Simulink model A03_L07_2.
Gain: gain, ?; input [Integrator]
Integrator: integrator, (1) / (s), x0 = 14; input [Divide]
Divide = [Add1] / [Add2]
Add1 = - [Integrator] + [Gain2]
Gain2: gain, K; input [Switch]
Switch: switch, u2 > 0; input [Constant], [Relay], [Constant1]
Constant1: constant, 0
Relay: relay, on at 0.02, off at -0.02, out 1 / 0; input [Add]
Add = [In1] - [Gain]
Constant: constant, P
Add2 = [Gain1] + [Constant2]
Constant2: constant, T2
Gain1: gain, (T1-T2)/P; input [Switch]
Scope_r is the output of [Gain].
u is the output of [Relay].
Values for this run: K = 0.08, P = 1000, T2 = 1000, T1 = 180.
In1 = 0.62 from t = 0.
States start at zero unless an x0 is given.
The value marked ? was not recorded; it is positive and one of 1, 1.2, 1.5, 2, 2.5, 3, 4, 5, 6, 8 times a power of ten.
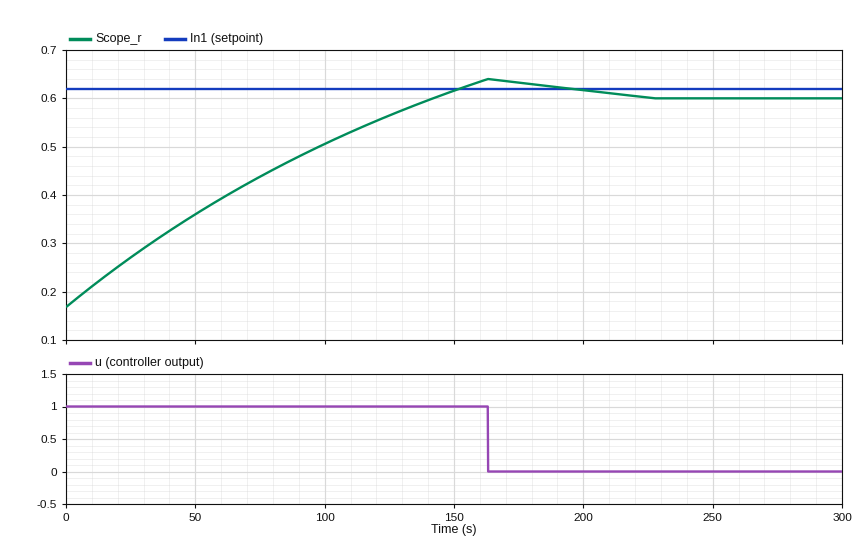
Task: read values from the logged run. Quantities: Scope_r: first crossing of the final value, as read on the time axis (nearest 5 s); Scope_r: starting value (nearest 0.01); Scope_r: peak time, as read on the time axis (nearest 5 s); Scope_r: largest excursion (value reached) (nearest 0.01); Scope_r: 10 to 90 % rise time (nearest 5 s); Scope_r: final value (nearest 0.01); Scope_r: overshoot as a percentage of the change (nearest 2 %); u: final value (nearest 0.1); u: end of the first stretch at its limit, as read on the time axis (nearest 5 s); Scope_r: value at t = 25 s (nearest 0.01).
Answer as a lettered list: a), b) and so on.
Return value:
a) 140 s
b) 0.17
c) 165 s
d) 0.64
e) 110 s
f) 0.60
g) 10 %
h) 0.0
i) 165 s
j) 0.27
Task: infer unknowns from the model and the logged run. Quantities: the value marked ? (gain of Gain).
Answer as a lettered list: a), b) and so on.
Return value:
a) 0.012
